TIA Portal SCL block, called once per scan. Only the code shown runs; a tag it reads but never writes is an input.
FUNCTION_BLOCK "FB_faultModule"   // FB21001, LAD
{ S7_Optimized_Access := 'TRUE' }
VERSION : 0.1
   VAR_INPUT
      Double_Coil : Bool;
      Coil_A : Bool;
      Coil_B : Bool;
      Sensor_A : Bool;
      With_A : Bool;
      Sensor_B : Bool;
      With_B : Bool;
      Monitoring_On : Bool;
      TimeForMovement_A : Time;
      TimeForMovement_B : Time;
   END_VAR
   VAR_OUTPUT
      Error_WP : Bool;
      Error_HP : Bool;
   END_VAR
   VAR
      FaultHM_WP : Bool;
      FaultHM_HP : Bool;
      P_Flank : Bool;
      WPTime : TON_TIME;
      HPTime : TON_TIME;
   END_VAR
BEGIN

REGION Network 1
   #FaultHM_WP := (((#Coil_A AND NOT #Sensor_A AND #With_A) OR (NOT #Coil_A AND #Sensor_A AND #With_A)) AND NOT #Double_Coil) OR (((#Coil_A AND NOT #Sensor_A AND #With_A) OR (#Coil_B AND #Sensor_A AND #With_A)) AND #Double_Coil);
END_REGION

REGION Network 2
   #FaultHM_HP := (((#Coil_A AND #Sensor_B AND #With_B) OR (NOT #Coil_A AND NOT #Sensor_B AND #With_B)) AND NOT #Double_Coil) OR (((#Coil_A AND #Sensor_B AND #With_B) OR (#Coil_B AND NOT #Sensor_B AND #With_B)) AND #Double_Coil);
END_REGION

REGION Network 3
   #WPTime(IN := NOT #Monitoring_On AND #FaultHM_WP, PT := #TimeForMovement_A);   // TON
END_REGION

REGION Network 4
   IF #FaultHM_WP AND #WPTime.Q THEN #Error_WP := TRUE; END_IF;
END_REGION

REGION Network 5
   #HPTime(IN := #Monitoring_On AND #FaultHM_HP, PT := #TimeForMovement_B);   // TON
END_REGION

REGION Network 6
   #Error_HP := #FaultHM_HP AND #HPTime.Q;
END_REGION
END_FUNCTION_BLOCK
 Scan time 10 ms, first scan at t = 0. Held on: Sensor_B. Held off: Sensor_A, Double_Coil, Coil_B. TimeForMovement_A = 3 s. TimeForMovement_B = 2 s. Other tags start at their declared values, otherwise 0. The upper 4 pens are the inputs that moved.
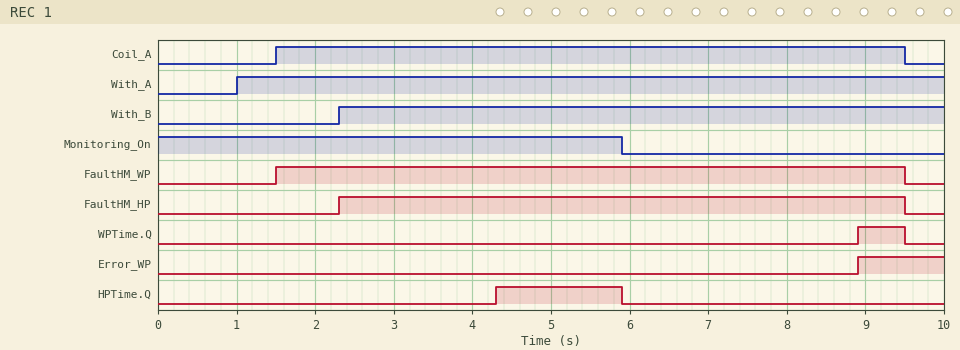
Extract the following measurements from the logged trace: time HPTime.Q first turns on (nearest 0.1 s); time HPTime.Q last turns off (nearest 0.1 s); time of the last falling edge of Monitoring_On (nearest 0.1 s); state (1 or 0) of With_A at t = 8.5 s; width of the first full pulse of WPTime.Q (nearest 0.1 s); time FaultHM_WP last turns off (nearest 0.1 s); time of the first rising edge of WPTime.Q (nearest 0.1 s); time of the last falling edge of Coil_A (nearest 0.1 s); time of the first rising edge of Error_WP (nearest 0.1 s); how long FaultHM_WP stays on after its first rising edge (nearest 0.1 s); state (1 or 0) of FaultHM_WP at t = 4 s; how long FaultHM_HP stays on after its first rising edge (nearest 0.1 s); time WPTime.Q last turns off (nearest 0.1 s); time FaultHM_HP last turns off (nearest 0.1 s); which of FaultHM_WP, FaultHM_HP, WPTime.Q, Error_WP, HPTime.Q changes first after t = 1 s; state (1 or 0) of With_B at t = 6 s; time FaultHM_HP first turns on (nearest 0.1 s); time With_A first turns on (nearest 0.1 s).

4.3 s
5.9 s
5.9 s
1
0.6 s
9.5 s
8.9 s
9.5 s
8.9 s
8.0 s
1
7.2 s
9.5 s
9.5 s
FaultHM_WP
1
2.3 s
1.0 s
